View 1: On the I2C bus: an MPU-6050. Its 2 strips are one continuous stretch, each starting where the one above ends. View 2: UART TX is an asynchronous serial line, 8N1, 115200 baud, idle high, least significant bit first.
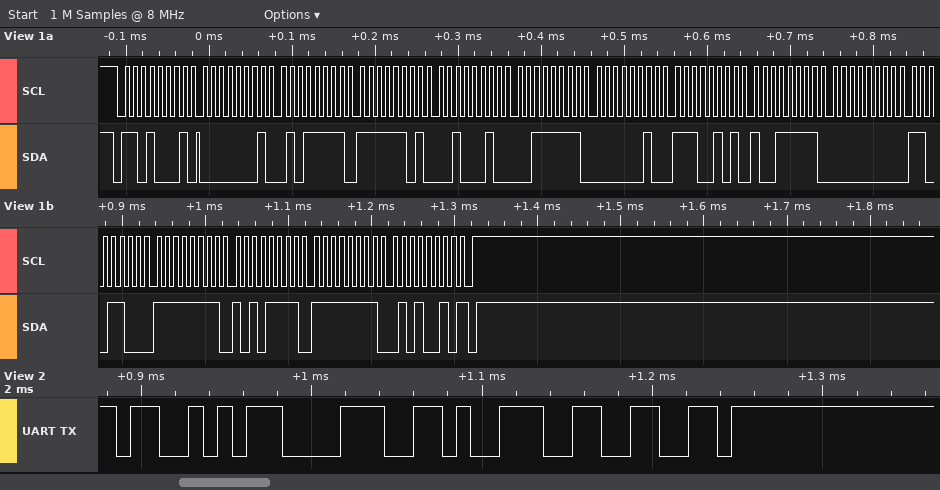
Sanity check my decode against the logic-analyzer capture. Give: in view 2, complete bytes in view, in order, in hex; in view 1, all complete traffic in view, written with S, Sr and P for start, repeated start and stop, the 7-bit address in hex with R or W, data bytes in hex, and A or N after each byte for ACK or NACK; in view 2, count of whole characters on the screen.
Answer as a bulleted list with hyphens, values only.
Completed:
- 53 38 39 66
- S 68R A 01 A 5F A FD A 22 A 3F A 02 A E5 A 9F A 00 A CC A FF A AF A FF A 52 N P
- 4
